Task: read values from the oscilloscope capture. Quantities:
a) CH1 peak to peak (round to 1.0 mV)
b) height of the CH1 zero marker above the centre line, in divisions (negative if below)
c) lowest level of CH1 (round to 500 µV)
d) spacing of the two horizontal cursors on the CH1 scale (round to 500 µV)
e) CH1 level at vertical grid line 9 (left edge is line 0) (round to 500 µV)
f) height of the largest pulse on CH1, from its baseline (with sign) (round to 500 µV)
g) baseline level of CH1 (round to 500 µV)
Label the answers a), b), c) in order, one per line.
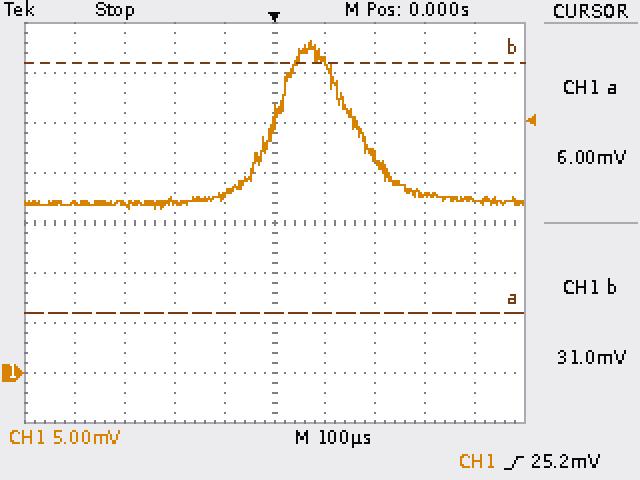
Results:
a) 17.0 mV
b) -3.0 div
c) 16.5 mV
d) 25.0 mV
e) 17.5 mV
f) +16.0 mV
g) 17.0 mV
